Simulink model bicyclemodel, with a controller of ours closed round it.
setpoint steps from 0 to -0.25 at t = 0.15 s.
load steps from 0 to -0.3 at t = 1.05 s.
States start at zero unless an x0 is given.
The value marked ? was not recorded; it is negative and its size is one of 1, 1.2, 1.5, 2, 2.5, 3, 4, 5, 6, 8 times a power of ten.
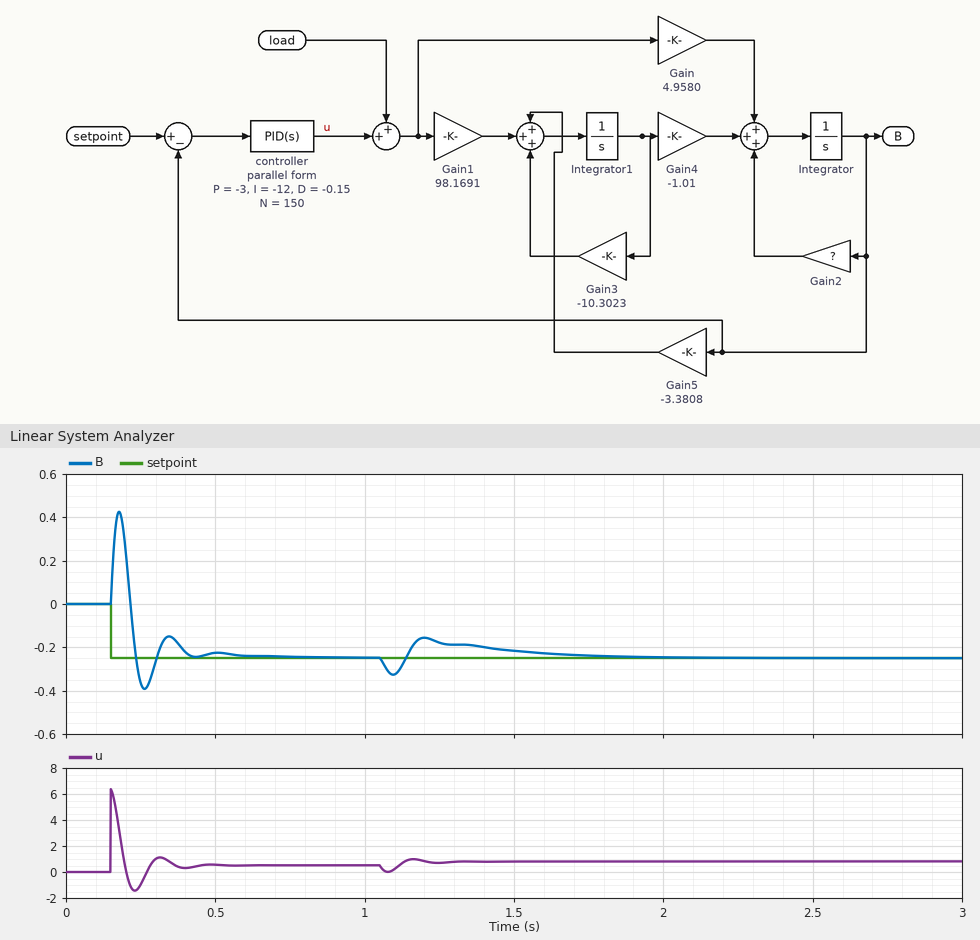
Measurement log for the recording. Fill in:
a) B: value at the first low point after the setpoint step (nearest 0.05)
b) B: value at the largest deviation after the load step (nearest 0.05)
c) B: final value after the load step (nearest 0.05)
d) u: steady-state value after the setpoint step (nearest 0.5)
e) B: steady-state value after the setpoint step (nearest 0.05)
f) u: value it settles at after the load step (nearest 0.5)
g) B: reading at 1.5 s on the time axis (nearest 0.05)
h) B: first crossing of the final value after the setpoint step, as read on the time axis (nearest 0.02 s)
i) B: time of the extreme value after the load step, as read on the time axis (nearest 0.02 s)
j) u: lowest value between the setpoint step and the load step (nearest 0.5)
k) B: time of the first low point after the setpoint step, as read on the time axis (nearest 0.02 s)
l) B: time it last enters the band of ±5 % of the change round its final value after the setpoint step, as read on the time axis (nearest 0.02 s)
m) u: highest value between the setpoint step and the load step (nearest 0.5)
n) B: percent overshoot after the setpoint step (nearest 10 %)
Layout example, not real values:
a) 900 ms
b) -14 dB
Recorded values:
a) -0.40
b) -0.15
c) -0.25
d) 0.5
e) -0.25
f) 1.0
g) -0.20
h) 0.24 s
i) 1.20 s
j) -1.5
k) 0.26 s
l) 0.58 s
m) 6.5
n) 60 %
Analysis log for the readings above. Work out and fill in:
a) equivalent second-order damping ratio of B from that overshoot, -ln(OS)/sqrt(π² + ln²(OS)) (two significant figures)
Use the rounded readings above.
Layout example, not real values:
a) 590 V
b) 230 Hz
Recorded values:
a) 0.16
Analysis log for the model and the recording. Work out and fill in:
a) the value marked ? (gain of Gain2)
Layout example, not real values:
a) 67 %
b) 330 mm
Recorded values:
a) -10
